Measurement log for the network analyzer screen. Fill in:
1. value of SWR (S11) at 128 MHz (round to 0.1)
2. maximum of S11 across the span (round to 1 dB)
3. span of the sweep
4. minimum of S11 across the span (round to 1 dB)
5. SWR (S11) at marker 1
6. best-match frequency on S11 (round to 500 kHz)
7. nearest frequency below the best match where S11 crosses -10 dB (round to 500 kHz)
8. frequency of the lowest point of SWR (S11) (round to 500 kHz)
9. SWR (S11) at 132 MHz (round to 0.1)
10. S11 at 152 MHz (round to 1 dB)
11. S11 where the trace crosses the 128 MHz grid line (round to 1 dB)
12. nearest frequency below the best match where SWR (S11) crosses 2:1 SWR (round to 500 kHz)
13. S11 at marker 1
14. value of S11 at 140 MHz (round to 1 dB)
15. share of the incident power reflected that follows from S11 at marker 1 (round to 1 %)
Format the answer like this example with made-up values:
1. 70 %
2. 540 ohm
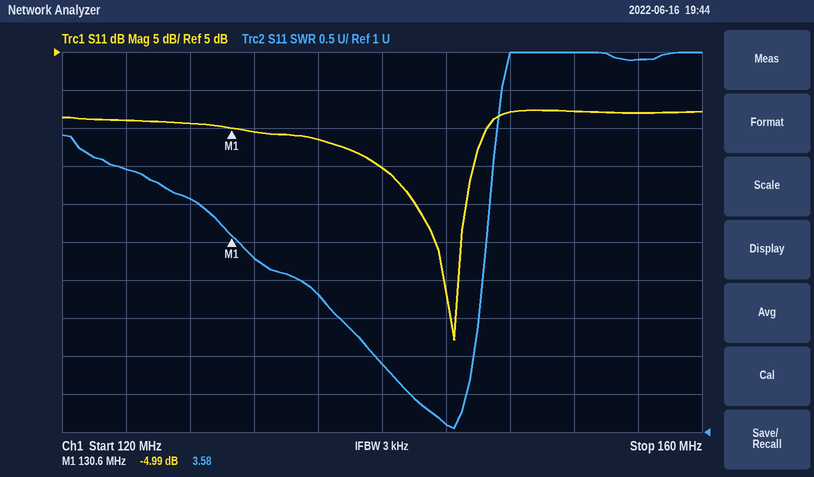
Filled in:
1. 4.1
2. -3 dB
3. 40 MHz
4. -33 dB
5. 3.58
6. 144.5 MHz
7. 140.0 MHz
8. 144.5 MHz
9. 3.3
10. -3 dB
11. -4 dB
12. 139.5 MHz
13. -4.99 dB
14. -10 dB
15. 32 %
